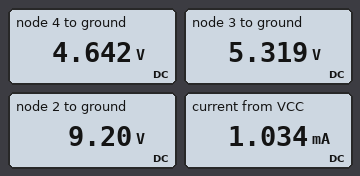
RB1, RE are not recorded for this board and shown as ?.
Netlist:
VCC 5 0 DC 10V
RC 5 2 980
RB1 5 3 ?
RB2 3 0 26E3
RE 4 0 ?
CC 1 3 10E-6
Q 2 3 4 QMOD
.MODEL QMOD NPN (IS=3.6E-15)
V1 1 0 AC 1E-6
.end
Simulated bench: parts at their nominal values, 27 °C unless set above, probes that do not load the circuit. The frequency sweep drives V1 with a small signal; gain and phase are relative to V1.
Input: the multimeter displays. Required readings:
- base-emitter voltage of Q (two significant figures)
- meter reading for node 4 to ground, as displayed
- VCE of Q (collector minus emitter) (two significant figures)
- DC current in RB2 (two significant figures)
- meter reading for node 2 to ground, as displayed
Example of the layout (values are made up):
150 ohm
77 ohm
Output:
680 mV
4.642 V
4.6 V
200 µA
9.20 V
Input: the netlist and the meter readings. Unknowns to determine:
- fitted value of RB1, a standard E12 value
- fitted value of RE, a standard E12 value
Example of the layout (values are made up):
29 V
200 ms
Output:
22 kΩ
5.6 kΩ
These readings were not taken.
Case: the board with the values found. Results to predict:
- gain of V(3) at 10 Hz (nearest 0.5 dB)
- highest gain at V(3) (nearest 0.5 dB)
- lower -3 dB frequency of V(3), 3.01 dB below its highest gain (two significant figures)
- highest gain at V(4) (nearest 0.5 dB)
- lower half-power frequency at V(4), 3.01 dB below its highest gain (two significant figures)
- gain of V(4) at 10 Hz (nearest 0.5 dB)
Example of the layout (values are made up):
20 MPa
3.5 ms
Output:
0 dB
0 dB
1.4 Hz
0 dB
1.4 Hz
0 dB
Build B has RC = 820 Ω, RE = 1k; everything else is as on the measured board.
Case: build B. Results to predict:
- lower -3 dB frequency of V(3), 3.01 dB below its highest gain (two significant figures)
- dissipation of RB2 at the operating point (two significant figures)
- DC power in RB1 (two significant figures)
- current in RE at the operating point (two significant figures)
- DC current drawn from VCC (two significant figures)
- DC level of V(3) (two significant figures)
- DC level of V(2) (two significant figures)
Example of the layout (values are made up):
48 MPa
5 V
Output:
1.5 Hz
930 µW
1.2 mW
4.2 mA
4.4 mA
4.9 V
6.6 V
